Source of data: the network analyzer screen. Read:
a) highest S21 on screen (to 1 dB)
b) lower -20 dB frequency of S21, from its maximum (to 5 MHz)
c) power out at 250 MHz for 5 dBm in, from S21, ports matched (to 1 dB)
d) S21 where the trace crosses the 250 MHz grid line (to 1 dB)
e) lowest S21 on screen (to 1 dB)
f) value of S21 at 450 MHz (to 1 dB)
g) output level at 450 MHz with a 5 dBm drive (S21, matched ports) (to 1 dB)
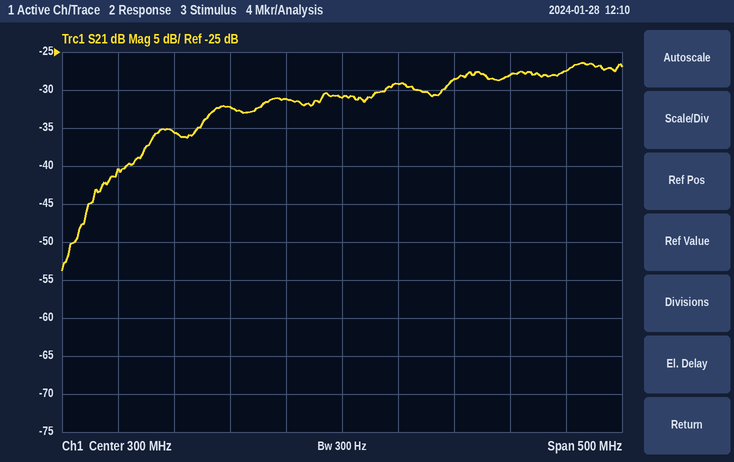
-26 dB
70 MHz
-26 dBm
-31 dB
-54 dB
-28 dB
-23 dBm
